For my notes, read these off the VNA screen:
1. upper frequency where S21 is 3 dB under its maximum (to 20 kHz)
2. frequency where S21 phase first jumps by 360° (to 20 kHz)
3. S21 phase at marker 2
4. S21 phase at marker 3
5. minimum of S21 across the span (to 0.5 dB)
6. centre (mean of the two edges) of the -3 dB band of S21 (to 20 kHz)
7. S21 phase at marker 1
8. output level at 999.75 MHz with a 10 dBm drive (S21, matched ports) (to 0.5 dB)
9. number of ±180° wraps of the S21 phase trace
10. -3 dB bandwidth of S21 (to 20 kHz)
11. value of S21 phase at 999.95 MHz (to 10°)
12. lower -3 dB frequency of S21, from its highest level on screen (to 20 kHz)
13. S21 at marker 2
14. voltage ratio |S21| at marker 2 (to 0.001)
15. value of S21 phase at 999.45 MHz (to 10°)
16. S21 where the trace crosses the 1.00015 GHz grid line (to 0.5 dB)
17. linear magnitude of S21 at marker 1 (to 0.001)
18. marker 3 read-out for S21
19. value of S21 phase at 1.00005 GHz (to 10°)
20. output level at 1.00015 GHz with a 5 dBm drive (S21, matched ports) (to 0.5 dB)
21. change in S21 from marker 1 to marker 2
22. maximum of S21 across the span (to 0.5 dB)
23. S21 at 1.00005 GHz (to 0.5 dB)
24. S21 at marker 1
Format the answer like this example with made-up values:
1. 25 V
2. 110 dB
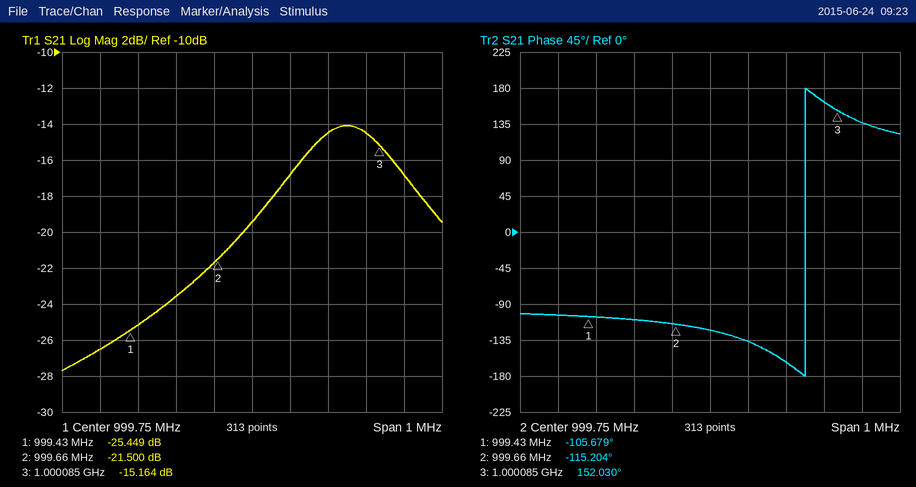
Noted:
1. 1.00016 GHz
2. 1.00000 GHz
3. -115.204°
4. 152.030°
5. -27.5 dB
6. 1.00000 GHz
7. -105.679°
8. -9.5 dBm
9. 1
10. 320 kHz
11. -160°
12. 999.84 MHz
13. -21.500 dB
14. 0.084
15. -110°
16. -17.0 dB
17. 0.053
18. -15.164 dB
19. 160°
20. -12.0 dBm
21. 3.949 dB
22. -14.0 dB
23. -14.5 dB
24. -25.449 dB
